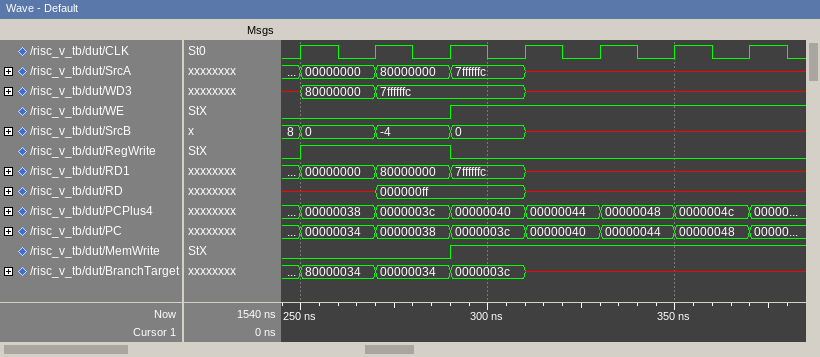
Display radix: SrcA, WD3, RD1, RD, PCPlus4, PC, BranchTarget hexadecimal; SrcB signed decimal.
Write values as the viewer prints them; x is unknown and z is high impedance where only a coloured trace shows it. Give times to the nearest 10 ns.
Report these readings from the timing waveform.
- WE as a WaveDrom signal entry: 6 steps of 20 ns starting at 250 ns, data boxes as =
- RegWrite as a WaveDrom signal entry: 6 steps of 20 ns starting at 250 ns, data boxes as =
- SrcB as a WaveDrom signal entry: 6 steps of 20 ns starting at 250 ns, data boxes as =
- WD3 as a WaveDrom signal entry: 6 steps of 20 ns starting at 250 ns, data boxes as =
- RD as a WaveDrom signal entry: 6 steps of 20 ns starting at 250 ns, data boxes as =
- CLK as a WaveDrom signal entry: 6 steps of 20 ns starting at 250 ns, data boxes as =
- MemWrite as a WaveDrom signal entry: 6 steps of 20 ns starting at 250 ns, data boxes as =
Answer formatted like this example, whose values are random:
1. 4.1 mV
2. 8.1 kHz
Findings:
1. {name: 'WE', wave: '0.1...'}
2. {name: 'RegWrite', wave: '1.0...'}
3. {name: 'SrcB', wave: '===x..', data: '0 -4 0'}
4. {name: 'WD3', wave: '==.x..', data: '80000000 7ffffffc'}
5. {name: 'RD', wave: 'x=.x..', data: '000000ff'}
6. {name: 'CLK', wave: 'p.....'}
7. {name: 'MemWrite', wave: '0.1...'}
